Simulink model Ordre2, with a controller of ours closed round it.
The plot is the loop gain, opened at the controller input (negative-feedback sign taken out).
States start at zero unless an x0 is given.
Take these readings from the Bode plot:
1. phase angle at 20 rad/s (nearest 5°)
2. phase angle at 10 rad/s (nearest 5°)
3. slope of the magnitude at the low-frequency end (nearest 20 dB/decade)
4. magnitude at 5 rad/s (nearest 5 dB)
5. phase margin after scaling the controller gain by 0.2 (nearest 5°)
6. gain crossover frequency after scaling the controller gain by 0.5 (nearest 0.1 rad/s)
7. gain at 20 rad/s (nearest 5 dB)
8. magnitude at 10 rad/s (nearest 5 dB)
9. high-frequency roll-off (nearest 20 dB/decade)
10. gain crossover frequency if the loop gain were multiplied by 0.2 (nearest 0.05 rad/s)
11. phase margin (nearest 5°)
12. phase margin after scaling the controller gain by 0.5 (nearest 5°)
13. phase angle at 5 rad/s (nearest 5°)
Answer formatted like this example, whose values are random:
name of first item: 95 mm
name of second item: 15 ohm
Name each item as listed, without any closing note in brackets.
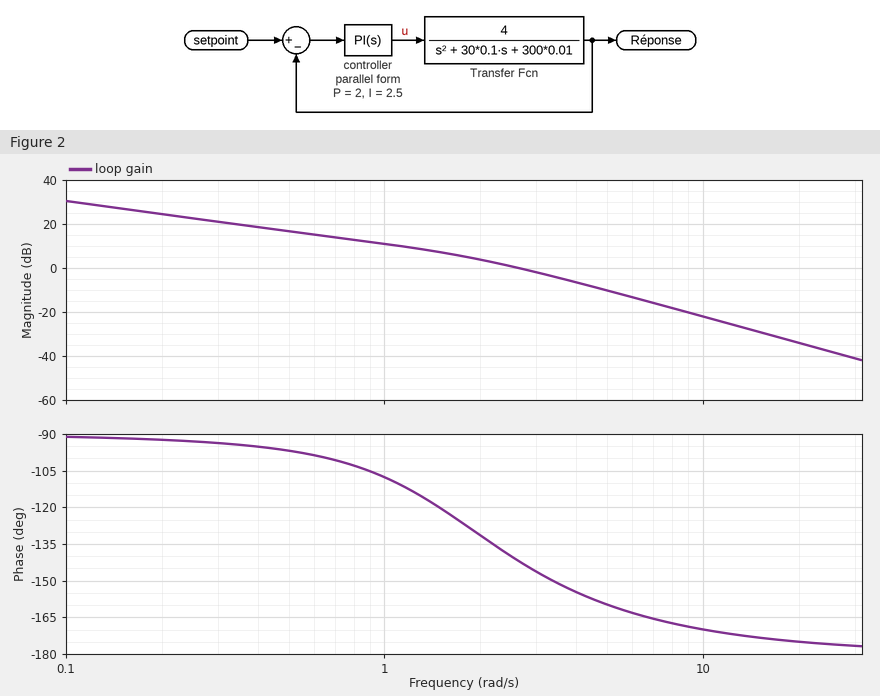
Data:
phase angle at 20 rad/s: -175°
phase angle at 10 rad/s: -170°
slope of the magnitude at the low-frequency end: -20 dB/decade
magnitude at 5 rad/s: -10 dB
phase margin after scaling the controller gain by 0.2: 80°
gain crossover frequency after scaling the controller gain by 0.5: 1.7 rad/s
gain at 20 rad/s: -35 dB
magnitude at 10 rad/s: -20 dB
high-frequency roll-off: -40 dB/decade
gain crossover frequency if the loop gain were multiplied by 0.2: 0.70 rad/s
phase margin: 40°
phase margin after scaling the controller gain by 0.5: 55°
phase angle at 5 rad/s: -160°
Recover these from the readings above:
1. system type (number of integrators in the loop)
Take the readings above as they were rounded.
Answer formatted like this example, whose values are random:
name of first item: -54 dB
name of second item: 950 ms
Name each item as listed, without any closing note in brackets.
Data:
system type: 1
